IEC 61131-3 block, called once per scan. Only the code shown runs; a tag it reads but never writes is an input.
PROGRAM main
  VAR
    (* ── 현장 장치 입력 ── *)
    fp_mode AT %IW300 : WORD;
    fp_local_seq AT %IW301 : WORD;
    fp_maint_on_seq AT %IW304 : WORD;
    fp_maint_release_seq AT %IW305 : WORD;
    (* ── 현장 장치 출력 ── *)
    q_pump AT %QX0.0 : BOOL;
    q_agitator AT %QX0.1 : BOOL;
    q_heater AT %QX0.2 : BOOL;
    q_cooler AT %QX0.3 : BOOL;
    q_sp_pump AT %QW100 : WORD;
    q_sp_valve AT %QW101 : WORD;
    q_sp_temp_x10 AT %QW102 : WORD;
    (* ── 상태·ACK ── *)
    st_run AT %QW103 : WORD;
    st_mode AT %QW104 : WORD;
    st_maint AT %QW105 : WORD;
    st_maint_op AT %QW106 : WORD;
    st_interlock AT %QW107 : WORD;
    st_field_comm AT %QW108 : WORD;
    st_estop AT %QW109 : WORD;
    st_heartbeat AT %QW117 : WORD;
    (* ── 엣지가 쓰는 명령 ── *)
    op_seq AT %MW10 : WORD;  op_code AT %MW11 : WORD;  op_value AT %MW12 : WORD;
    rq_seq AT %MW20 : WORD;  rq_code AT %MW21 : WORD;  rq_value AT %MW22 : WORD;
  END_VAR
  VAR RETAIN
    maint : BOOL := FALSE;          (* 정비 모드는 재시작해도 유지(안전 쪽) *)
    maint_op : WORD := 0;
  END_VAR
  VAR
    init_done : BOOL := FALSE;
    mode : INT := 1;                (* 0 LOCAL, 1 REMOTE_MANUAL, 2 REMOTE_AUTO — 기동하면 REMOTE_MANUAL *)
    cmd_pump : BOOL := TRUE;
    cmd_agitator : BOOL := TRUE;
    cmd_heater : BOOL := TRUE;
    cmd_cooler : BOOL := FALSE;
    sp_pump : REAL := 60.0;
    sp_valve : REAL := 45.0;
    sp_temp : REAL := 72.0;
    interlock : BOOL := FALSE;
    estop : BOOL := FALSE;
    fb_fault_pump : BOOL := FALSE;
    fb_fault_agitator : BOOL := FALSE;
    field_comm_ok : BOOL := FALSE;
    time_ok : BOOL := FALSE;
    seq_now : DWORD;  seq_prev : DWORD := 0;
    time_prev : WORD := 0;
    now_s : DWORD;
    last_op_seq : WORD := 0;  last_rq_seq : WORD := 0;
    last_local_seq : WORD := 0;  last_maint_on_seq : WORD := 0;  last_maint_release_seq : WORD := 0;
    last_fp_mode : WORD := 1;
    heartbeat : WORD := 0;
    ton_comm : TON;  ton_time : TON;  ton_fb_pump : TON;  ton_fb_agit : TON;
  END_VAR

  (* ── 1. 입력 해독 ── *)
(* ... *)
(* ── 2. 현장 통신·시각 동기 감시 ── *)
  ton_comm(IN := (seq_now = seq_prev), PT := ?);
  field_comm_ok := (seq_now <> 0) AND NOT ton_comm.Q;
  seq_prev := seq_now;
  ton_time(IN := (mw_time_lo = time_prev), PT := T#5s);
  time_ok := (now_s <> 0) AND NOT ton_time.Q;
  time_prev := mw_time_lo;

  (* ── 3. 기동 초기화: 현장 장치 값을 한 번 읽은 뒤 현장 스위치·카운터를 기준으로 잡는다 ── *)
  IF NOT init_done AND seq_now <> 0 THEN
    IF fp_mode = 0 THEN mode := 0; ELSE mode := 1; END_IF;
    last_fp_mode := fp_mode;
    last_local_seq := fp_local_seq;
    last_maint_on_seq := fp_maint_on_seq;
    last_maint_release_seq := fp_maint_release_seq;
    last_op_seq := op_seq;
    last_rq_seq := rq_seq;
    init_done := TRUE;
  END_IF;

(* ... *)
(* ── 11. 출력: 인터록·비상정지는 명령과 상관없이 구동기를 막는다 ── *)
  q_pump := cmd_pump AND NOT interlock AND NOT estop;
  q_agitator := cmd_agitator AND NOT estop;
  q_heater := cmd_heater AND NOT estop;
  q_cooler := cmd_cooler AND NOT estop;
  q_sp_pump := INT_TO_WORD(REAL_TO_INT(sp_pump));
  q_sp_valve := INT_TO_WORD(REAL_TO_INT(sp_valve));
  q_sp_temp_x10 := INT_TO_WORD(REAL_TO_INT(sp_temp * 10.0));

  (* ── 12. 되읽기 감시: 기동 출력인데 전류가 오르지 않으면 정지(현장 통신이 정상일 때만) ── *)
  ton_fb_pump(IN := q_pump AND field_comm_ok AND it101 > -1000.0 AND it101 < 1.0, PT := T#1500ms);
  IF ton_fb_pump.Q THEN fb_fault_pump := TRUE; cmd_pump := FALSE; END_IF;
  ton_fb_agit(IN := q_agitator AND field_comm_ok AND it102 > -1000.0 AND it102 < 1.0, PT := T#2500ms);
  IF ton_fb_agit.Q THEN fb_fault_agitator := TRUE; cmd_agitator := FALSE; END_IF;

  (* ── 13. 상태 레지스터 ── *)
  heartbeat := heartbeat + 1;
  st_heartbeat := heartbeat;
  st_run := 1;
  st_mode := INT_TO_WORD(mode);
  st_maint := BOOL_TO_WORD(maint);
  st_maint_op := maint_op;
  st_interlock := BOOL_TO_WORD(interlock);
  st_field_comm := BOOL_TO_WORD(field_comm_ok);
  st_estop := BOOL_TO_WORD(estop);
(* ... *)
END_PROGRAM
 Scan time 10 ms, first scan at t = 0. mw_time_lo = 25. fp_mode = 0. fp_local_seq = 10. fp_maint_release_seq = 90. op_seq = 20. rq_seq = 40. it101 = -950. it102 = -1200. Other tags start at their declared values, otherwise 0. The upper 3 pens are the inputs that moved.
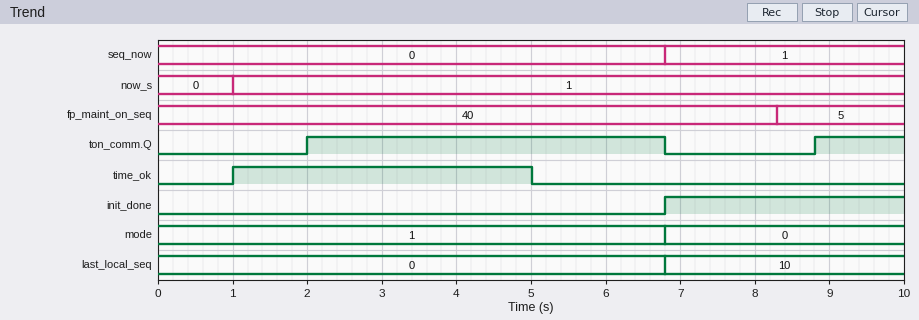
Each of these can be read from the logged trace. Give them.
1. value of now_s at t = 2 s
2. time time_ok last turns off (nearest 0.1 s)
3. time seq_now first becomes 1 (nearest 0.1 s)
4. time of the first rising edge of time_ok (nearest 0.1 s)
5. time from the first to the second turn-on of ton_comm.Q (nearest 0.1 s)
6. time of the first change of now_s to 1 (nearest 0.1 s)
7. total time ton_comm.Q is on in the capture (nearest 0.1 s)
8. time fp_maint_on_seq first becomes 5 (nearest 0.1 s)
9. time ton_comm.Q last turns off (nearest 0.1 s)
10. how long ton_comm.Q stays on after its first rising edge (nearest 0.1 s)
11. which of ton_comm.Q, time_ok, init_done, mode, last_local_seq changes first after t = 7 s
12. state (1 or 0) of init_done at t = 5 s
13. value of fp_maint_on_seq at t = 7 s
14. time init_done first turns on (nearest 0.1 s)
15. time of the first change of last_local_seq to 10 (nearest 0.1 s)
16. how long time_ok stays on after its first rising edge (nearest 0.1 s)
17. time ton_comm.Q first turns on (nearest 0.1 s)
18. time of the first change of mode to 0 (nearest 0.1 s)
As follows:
1
5.0 s
6.8 s
1.0 s
6.8 s
1.0 s
6.0 s
8.3 s
6.8 s
4.8 s
ton_comm.Q
0
40
6.8 s
6.8 s
4.0 s
2.0 s
6.8 s
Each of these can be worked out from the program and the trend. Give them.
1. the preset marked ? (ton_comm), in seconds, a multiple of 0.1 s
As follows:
2.0 s
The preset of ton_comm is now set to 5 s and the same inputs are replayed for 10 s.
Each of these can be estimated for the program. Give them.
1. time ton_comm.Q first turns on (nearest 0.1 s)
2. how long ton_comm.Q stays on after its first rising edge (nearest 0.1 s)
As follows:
5.0 s
1.8 s
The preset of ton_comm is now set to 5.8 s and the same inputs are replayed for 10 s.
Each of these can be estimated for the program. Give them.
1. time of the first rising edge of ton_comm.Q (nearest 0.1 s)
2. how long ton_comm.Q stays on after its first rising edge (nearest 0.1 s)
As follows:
5.8 s
1.0 s
